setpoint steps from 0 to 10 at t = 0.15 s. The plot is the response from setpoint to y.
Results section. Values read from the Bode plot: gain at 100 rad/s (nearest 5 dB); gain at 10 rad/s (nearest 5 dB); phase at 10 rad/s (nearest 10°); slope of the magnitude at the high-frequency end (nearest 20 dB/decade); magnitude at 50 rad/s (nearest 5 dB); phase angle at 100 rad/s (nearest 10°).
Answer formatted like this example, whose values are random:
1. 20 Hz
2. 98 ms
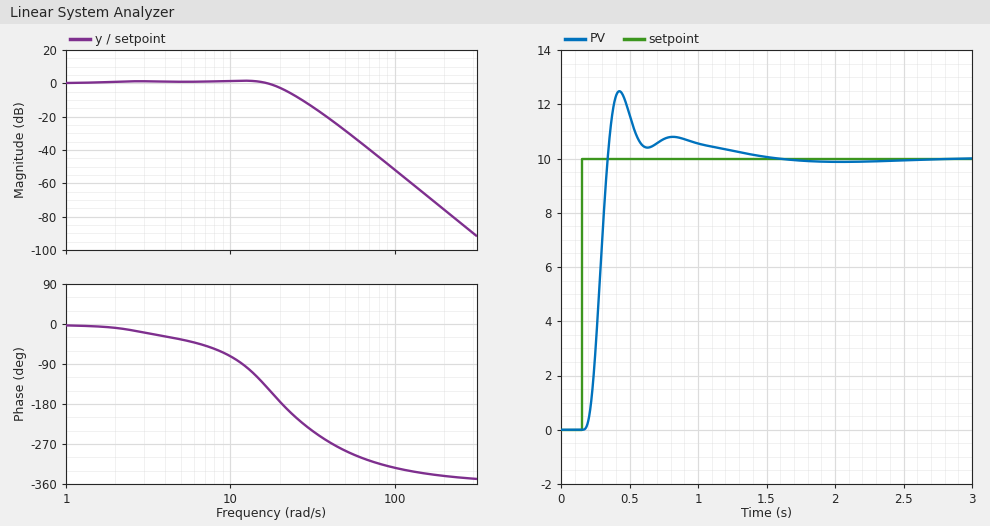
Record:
1. -50 dB
2. 0 dB
3. -70°
4. -80 dB/decade
5. -30 dB
6. -320°
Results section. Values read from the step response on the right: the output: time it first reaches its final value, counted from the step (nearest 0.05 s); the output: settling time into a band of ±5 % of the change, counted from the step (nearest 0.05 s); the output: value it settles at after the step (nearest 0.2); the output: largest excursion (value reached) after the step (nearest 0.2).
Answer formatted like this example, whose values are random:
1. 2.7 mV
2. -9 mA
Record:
1. 0.20 s
2. 0.90 s
3. 10.0
4. 12.4
